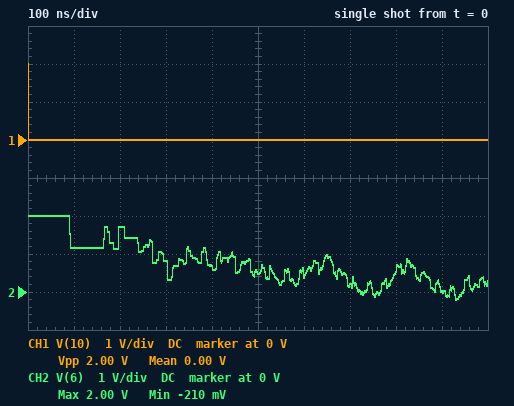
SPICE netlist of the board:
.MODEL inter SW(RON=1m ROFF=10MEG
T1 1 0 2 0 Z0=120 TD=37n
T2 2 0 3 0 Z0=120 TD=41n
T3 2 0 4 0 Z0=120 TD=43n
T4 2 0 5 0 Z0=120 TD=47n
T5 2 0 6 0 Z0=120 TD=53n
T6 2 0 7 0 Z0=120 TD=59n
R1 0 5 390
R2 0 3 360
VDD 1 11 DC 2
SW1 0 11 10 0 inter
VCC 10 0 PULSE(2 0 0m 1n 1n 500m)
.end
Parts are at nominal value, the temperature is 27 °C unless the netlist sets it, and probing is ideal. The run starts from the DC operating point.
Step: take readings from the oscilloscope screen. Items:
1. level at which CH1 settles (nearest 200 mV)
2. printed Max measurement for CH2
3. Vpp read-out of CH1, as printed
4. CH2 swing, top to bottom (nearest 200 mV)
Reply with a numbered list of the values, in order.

1. 0 V
2. 2.00 V
3. 2.00 V
4. 2.2 V
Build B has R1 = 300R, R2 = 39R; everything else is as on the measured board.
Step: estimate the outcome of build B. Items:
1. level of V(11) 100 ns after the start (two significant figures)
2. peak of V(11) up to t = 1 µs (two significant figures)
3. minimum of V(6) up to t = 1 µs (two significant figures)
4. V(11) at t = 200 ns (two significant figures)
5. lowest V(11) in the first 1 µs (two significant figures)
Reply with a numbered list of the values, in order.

1. 2.3 V
2. 5.2 V
3. -3.8 V
4. -8.4 V
5. -9.0 V
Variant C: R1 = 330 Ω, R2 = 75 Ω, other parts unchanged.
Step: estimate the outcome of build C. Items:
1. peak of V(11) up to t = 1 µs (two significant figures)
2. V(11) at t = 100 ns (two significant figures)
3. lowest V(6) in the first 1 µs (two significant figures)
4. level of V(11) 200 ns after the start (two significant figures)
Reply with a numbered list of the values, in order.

1. 1.8 V
2. 1.3 V
3. -1.9 V
4. -5.0 V
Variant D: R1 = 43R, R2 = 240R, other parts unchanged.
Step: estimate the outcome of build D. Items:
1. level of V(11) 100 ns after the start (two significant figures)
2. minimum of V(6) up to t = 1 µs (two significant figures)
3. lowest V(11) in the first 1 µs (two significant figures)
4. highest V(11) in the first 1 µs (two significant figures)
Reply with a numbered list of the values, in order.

1. 2.2 V
2. -3.5 V
3. -7.8 V
4. 3.6 V
